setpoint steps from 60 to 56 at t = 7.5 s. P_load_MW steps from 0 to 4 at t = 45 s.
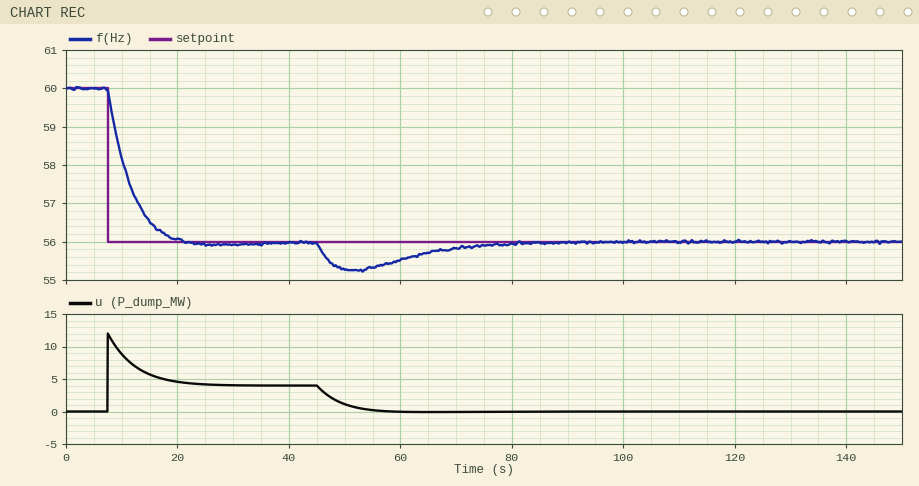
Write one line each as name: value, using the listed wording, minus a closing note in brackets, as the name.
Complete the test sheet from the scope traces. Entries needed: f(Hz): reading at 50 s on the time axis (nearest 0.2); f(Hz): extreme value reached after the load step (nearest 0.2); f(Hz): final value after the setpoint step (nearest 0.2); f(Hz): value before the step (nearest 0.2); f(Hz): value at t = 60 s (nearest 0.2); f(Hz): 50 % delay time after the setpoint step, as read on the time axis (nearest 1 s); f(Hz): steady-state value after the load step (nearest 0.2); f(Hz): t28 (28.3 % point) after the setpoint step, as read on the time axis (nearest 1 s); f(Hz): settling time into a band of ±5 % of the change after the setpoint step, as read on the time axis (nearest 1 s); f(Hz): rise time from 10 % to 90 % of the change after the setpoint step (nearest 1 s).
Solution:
f(Hz): reading at 50 s on the time axis: 55.2
f(Hz): extreme value reached after the load step: 55.2
f(Hz): final value after the setpoint step: 56.0
f(Hz): value before the step: 60.0
f(Hz): value at t = 60 s: 55.6
f(Hz): 50 % delay time after the setpoint step, as read on the time axis: 10 s
f(Hz): steady-state value after the load step: 56.0
f(Hz): t28 (28.3 % point) after the setpoint step, as read on the time axis: 9 s
f(Hz): settling time into a band of ±5 % of the change after the setpoint step, as read on the time axis: 18 s
f(Hz): rise time from 10 % to 90 % of the change after the setpoint step: 8 s
